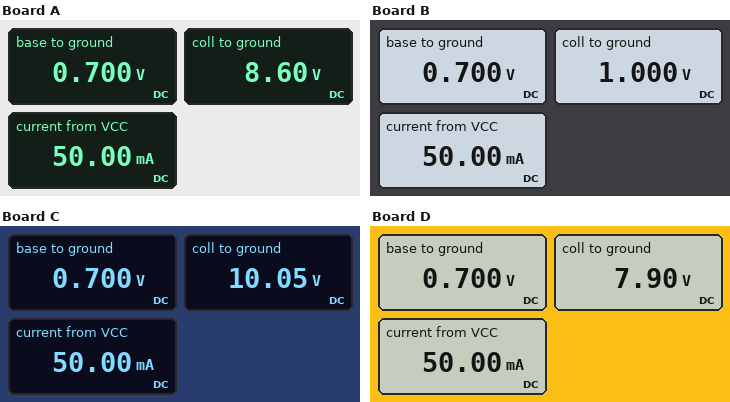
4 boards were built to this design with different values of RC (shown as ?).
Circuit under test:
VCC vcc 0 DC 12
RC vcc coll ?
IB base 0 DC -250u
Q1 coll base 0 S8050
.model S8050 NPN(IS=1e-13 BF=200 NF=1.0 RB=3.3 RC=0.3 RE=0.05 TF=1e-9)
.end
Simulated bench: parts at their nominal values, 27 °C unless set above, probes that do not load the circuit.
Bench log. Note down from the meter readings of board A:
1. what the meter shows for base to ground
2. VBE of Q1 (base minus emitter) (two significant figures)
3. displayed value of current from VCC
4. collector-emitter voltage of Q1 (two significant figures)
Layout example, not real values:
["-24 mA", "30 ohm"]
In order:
["0.700 V", "700 mV", "50.00 mA", "8.6 V"]
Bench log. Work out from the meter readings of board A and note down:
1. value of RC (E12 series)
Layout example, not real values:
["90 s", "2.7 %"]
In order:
["68 Ω"]
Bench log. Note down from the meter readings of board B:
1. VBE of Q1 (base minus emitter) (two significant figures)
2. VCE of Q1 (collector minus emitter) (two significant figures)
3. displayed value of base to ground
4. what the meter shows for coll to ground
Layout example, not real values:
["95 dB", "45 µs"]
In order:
["700 mV", "1.0 V", "0.700 V", "1.000 V"]
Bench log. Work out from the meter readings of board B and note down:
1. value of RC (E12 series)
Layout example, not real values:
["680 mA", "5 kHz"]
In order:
["220 Ω"]
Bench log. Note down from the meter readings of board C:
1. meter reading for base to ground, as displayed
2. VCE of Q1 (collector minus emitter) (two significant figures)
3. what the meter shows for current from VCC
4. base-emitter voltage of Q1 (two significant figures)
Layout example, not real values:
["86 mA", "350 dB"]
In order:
["0.700 V", "10 V", "50.00 mA", "700 mV"]
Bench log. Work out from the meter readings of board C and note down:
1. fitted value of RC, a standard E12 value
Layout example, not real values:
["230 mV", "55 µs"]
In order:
["39 Ω"]
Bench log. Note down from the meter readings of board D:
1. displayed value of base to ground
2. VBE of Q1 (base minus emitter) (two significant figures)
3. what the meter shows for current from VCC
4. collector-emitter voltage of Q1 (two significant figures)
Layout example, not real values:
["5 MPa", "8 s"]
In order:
["0.700 V", "700 mV", "50.00 mA", "7.9 V"]
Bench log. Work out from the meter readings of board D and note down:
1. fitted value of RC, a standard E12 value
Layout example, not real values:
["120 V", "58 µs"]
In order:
["82 Ω"]
